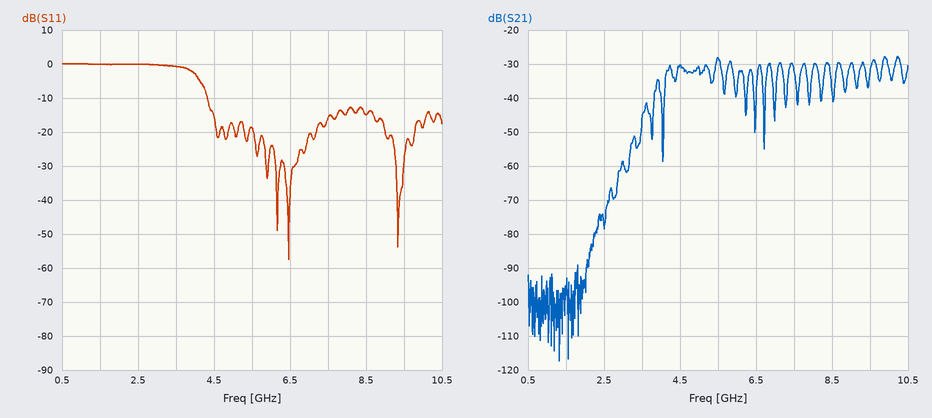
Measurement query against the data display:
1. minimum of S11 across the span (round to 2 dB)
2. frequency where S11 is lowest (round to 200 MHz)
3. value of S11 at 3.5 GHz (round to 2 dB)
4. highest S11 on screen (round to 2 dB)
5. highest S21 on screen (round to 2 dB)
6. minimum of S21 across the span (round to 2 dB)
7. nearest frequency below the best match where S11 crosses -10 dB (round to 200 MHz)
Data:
-58 dB
6.4 GHz
0 dB
0 dB
-28 dB
-118 dB
4.4 GHz
